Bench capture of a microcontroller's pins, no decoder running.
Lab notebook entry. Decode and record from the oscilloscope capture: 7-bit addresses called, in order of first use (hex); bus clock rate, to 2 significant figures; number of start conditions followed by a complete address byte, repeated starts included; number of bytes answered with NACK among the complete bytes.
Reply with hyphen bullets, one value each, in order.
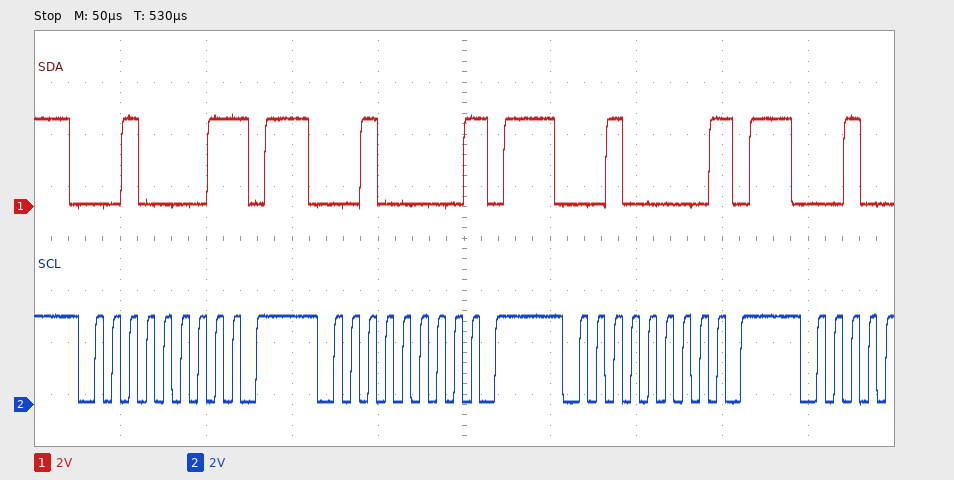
- 0x10
- 100 kHz
- 3
- 3
